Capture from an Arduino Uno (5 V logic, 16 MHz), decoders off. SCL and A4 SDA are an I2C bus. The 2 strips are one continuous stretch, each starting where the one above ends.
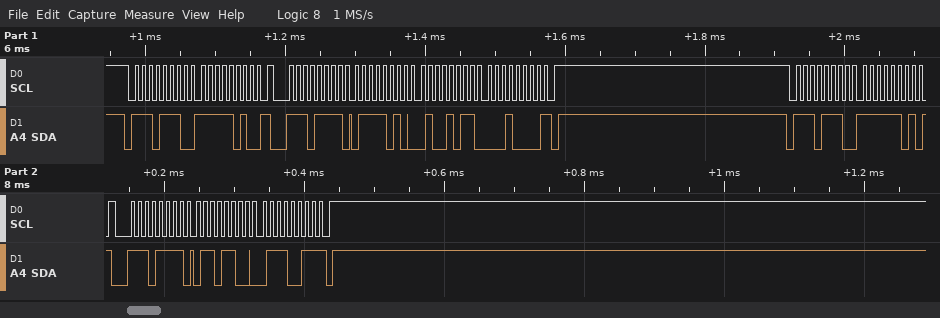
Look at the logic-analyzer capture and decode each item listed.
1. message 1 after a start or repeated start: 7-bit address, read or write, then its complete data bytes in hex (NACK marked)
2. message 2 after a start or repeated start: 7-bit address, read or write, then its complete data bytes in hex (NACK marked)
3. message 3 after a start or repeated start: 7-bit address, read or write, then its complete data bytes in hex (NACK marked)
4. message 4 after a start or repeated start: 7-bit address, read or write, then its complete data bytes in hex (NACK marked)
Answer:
0x77 write: FA
0x77 read: 7A 4B 10 NACK
0x77 write: FD
0x77 read: 6C 73 NACK
